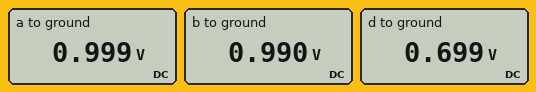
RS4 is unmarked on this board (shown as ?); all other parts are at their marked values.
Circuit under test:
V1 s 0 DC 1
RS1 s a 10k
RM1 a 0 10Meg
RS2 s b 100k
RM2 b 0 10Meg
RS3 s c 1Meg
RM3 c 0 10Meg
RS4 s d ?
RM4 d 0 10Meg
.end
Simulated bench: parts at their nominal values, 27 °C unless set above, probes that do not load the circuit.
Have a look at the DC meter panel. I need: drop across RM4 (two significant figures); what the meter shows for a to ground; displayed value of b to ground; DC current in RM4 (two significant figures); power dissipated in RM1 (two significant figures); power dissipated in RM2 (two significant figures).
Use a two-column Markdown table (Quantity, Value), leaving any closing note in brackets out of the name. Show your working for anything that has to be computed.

| Quantity | Value |
|---|---|
| drop across RM4 | 699 mV = 700 mV |
| what the meter shows for a to ground | 0.999 V |
| displayed value of b to ground | 0.990 V |
| DC current in RM4 | (699 mV) / 10 MΩ = 70 nA |
| power dissipated in RM1 | (999 mV)^2 / 10 MΩ = 100 nW |
| power dissipated in RM2 | (990 mV)^2 / 10 MΩ = 98 nW |
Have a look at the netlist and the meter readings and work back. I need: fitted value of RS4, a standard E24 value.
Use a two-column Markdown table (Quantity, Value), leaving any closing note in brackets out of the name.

| Quantity | Value |
|---|---|
| fitted value of RS4, a standard E24 value | 4.3 MΩ |
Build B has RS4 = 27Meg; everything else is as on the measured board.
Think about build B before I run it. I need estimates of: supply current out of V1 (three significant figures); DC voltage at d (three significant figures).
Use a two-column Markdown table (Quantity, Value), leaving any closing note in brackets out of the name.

| Quantity | Value |
|---|---|
| supply current out of V1 | 317 nA |
| DC voltage at d | 270 mV |
